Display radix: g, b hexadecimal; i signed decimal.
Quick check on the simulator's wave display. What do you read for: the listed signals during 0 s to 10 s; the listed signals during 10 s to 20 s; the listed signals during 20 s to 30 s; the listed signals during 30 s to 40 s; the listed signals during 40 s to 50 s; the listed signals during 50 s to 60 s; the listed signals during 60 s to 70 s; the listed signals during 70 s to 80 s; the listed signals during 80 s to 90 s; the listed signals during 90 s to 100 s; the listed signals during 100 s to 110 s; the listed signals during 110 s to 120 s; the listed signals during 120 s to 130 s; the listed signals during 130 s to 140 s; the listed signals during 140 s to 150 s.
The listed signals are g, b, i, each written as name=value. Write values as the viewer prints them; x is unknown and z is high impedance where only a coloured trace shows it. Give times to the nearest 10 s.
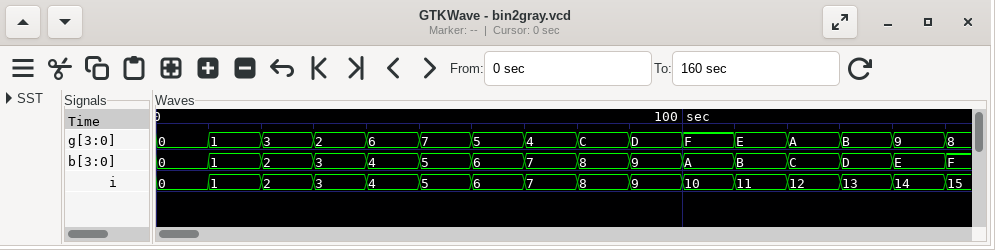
g=0, b=0, i=0
g=1, b=1, i=1
g=3, b=2, i=2
g=2, b=3, i=3
g=6, b=4, i=4
g=7, b=5, i=5
g=5, b=6, i=6
g=4, b=7, i=7
g=C, b=8, i=8
g=D, b=9, i=9
g=F, b=A, i=10
g=E, b=B, i=11
g=A, b=C, i=12
g=B, b=D, i=13
g=9, b=E, i=14
